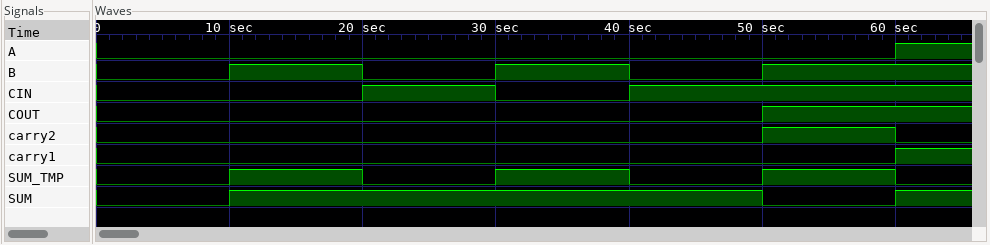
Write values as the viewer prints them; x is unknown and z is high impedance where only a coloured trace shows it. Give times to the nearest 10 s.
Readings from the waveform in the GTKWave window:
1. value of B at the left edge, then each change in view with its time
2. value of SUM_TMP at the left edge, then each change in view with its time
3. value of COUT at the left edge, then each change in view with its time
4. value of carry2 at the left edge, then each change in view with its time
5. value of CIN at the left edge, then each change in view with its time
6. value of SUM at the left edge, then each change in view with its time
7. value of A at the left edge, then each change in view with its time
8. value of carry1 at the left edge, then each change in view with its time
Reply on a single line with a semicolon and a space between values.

0, 1 at 10 s, 0 at 20 s, 1 at 30 s, 0 at 40 s, 1 at 50 s; 0, 1 at 10 s, 0 at 20 s, 1 at 30 s, 0 at 40 s, 1 at 50 s, 0 at 60 s; 0, 1 at 50 s; 0, 1 at 50 s, 0 at 60 s; 0, 1 at 20 s, 0 at 30 s, 1 at 40 s; 0, 1 at 10 s, 0 at 50 s, 1 at 60 s; 0, 1 at 60 s; 0, 1 at 60 s
